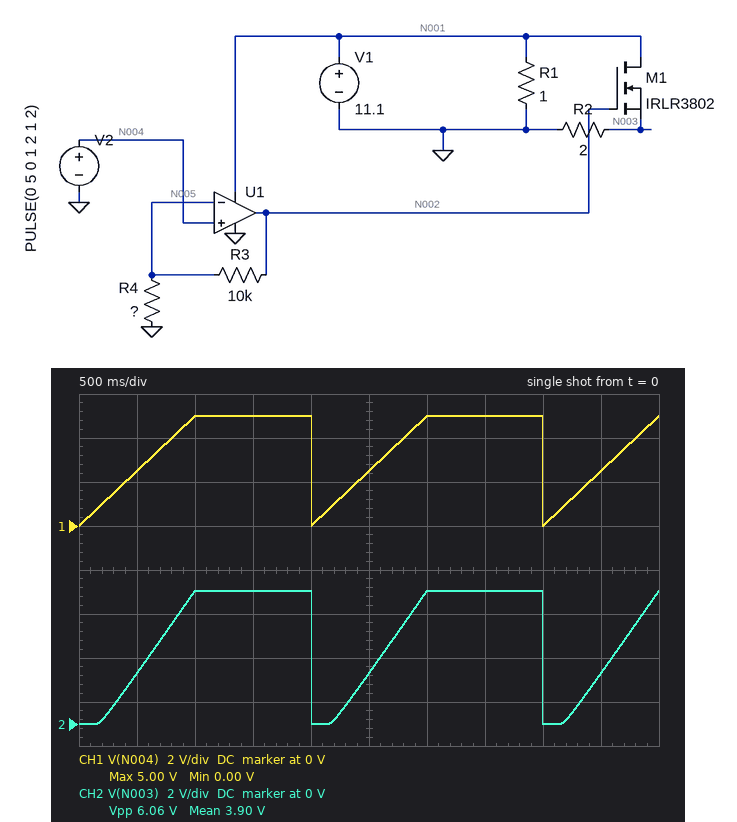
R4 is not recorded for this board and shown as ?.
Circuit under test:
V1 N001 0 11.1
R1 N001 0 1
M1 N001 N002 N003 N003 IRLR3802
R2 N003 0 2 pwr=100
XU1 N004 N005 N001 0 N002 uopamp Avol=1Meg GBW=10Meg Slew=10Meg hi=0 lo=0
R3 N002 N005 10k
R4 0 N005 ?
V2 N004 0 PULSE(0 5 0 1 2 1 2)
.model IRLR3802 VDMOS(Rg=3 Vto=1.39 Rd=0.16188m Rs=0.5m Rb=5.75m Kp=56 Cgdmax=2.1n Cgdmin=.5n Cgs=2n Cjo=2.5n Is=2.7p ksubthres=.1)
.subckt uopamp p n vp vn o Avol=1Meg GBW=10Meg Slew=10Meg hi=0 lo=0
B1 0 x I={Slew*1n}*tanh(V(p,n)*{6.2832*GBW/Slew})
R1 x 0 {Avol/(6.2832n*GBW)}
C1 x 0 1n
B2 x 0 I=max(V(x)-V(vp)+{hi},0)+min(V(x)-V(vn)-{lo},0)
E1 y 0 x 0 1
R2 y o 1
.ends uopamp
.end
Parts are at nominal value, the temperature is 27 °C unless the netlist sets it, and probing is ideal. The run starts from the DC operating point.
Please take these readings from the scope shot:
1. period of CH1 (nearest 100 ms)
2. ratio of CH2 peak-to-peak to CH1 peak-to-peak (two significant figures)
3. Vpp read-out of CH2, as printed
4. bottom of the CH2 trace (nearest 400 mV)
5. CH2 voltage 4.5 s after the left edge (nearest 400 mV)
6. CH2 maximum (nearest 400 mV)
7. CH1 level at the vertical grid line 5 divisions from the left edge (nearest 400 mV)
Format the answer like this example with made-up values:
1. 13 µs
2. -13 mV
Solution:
1. 2.0 s
2. 1.2
3. 6.06 V
4. 0 V
5. 2.4 V
6. 6.0 V
7. 2.4 V
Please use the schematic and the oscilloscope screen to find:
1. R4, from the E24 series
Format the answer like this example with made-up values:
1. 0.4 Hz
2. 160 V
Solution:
1. 18 kΩ
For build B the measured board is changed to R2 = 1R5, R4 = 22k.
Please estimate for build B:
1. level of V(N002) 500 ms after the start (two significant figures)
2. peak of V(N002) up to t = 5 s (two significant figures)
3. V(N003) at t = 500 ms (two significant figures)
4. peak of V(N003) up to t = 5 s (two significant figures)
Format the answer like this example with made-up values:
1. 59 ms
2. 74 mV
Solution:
1. 3.6 V
2. 7.3 V
3. 2.0 V
4. 5.5 V
